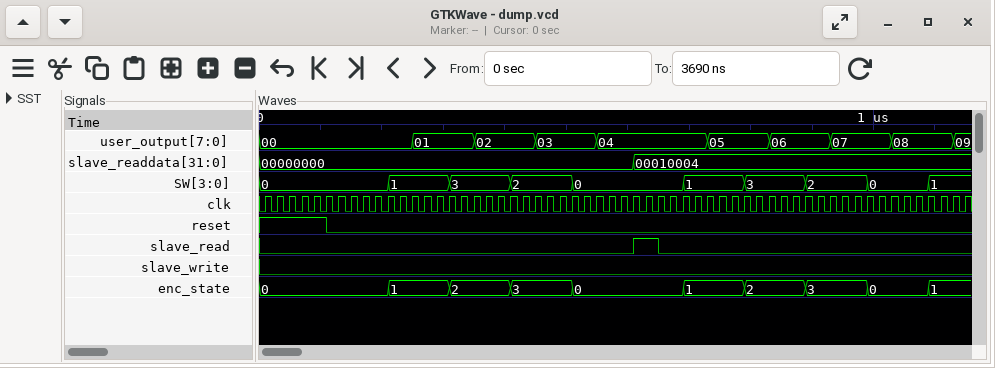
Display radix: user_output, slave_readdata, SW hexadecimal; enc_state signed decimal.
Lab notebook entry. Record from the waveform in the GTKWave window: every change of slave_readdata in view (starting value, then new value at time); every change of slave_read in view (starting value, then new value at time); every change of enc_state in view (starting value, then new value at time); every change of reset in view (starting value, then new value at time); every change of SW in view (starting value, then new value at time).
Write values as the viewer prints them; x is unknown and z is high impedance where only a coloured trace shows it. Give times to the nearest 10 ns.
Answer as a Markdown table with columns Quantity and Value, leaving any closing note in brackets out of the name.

| Quantity | Value |
|---|---|
| every change of slave_readdata in view | 00000000, 00010004 at 610 ns |
| every change of slave_read in view | 0, 1 at 610 ns, 0 at 650 ns |
| every change of enc_state in view | 0, 1 at 210 ns, 2 at 310 ns, 3 at 410 ns, 0 at 510 ns, 1 at 690 ns, 2 at 790 ns, 3 at 890 ns, 0 at 990 ns, 1 at 1090 ns |
| every change of reset in view | 1, 0 at 110 ns |
| every change of SW in view | 0, 1 at 210 ns, 3 at 310 ns, 2 at 410 ns, 0 at 510 ns, 1 at 690 ns, 3 at 790 ns, 2 at 890 ns, 0 at 990 ns, 1 at 1090 ns |
